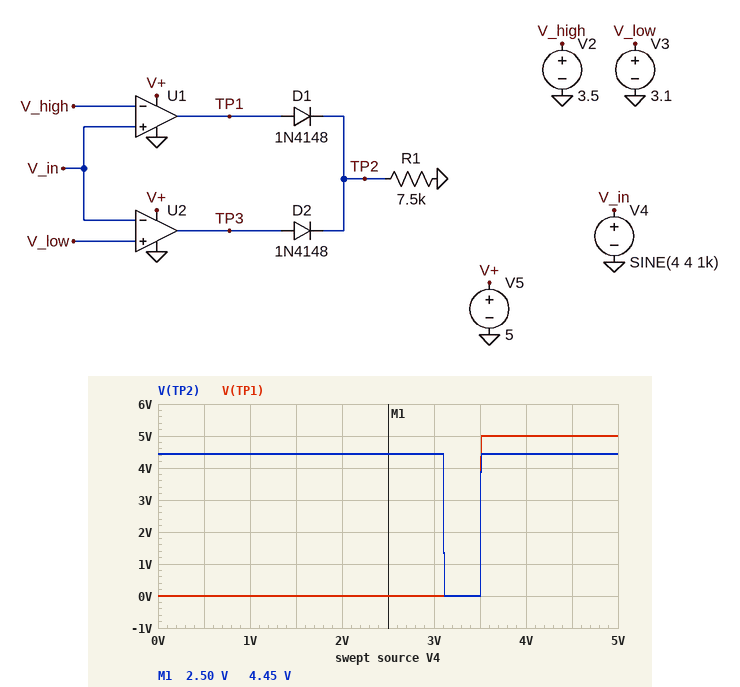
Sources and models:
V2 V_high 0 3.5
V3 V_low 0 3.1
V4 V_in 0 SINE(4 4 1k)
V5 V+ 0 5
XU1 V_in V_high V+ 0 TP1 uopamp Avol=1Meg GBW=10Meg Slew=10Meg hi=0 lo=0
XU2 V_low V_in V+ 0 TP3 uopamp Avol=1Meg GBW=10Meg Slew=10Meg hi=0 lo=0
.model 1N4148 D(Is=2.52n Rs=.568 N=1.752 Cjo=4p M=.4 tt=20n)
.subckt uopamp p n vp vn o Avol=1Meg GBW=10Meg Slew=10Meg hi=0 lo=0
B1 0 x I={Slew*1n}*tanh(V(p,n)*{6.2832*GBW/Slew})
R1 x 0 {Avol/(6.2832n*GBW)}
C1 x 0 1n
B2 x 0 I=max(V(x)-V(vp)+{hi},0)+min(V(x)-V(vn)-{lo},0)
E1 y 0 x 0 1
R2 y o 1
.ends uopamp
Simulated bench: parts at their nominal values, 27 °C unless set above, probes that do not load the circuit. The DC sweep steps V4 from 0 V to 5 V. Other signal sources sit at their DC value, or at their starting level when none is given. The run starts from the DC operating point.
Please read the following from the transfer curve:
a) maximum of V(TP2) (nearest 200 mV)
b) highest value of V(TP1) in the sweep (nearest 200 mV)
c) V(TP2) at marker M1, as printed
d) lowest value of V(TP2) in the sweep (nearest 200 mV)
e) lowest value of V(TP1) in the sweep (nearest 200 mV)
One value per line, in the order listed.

4.4 V
5.0 V
4.45 V
0 V
0 V
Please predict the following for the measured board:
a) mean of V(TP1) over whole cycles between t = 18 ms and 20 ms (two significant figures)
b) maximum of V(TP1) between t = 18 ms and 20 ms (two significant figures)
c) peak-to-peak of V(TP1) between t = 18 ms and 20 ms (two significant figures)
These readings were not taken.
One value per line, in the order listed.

2.7 V
5.0 V
5.0 V
